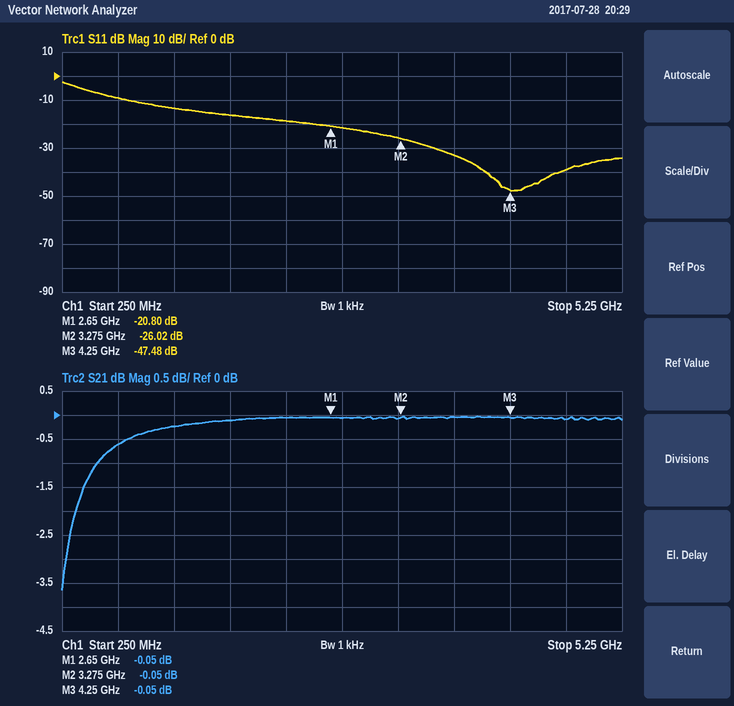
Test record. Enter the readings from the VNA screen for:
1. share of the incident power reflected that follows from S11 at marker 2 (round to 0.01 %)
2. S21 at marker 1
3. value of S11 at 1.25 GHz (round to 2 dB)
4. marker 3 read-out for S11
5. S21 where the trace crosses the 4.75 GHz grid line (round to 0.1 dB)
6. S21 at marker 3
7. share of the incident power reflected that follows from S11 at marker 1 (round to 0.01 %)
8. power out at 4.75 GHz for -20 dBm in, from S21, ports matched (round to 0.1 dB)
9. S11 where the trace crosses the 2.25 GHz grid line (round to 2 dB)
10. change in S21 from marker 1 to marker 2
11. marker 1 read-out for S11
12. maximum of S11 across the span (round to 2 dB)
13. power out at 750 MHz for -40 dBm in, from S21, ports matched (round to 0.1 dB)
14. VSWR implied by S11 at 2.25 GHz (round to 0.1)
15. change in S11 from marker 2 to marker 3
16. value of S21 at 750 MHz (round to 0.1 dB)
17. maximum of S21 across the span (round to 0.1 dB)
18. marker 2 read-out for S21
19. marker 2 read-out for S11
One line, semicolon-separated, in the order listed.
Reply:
0.25 %; -0.05 dB; -14 dB; -47.48 dB; -0.1 dB; -0.05 dB; 0.83 %; -20.1 dBm; -18 dB; 0.00 dB; -20.80 dB; -2 dB; -40.6 dBm; 1.3; -21.46 dB; -0.6 dB; 0.0 dB; -0.05 dB; -26.02 dB
